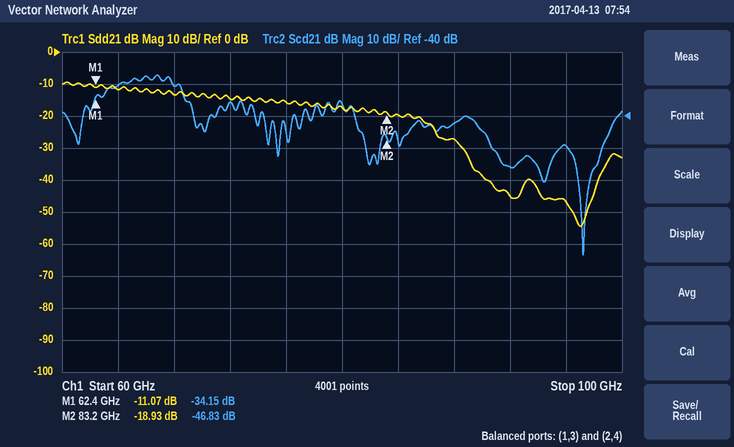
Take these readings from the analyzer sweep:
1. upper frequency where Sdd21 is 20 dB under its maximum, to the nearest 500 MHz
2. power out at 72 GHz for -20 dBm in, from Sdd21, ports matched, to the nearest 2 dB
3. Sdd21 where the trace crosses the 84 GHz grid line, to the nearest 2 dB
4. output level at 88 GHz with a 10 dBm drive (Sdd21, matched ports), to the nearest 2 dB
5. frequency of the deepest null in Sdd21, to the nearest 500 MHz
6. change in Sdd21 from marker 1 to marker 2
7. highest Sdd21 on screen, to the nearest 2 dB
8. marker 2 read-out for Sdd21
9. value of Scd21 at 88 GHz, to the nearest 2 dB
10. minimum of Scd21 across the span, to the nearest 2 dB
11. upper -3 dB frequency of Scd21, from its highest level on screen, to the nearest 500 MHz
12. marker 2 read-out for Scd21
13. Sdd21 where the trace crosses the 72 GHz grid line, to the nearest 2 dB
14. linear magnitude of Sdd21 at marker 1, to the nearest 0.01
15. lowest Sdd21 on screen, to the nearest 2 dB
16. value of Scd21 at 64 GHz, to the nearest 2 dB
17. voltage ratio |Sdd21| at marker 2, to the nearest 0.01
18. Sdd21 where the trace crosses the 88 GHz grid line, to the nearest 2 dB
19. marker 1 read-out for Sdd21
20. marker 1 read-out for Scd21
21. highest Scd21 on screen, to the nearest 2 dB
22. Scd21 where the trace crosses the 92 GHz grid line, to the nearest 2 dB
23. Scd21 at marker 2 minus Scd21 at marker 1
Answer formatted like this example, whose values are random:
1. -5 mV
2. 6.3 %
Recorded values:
1. 88.5 GHz
2. -34 dBm
3. -20 dB
4. -18 dBm
5. 97.0 GHz
6. -7.86 dB
7. -10 dB
8. -18.93 dB
9. -42 dB
10. -84 dB
11. 68.0 GHz
12. -46.83 dB
13. -14 dB
14. 0.28
15. -54 dB
16. -30 dB
17. 0.11
18. -28 dB
19. -11.07 dB
20. -34.15 dB
21. -28 dB
22. -56 dB
23. -12.68 dB
